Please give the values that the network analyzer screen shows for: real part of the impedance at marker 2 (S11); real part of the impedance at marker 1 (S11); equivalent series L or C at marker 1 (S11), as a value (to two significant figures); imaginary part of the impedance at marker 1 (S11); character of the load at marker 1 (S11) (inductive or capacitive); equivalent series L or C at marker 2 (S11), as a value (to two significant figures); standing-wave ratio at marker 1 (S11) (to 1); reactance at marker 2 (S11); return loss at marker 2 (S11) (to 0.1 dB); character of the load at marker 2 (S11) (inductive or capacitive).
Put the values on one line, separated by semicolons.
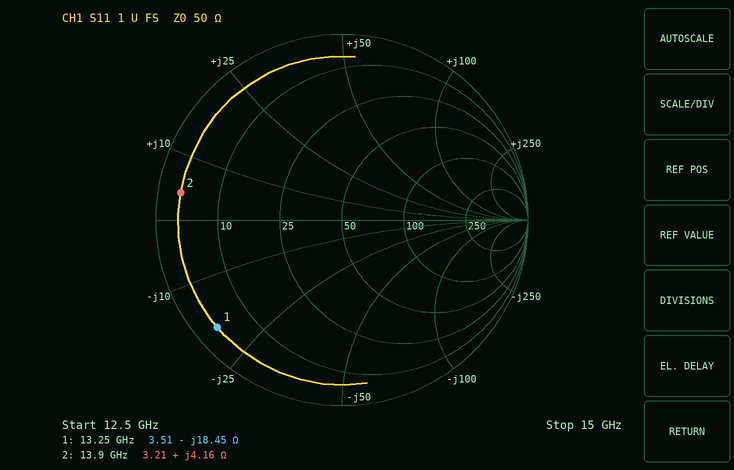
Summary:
3.21 Ω; 3.51 Ω; 650 fF; -18.45 Ω; capacitive; 48 pH; 16; +4.16 Ω; 1.1 dB; inductive
